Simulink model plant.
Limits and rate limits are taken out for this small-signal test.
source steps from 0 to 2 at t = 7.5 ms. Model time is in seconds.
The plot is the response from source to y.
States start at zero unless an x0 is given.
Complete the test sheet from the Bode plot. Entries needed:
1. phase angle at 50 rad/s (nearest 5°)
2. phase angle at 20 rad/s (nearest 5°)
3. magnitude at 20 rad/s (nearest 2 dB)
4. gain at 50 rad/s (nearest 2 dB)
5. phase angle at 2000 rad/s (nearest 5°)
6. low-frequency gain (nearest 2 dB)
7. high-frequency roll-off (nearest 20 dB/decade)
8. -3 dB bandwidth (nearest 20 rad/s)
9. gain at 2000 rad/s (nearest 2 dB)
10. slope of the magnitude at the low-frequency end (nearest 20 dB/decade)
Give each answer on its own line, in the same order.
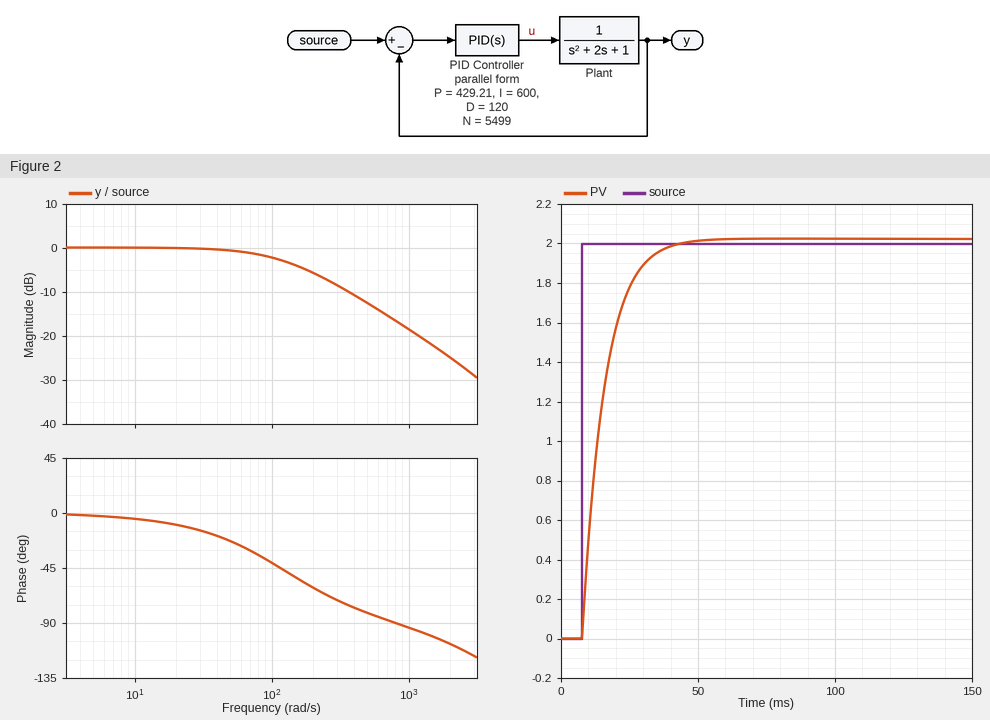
-25°
-10°
0 dB
0 dB
-105°
0 dB
-20 dB/decade
120 rad/s
-24 dB
0 dB/decade
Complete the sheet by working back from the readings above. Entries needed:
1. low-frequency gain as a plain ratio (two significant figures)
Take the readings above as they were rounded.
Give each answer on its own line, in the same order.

1.0
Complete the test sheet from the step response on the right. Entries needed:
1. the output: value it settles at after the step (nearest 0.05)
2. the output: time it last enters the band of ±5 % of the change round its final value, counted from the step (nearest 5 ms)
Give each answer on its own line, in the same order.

2.00
25 ms
